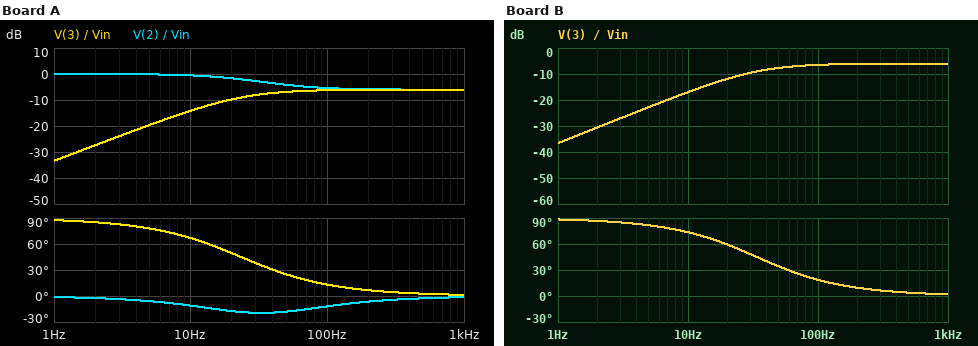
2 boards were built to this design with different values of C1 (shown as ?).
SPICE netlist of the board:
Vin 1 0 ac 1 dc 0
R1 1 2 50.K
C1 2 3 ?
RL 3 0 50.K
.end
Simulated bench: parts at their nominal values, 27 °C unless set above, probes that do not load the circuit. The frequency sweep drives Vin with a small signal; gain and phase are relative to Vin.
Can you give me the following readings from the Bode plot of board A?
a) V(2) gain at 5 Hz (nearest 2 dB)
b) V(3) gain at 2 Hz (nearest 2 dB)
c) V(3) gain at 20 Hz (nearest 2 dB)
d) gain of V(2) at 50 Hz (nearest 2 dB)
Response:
0 dB
-28 dB
-10 dB
-4 dB
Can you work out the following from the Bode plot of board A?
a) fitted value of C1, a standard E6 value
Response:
68 nF
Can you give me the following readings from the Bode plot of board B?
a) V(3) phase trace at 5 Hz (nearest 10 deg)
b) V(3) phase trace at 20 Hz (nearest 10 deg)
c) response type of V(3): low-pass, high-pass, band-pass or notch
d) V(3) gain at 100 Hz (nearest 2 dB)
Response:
80 deg
60 deg
high-pass
-6 dB
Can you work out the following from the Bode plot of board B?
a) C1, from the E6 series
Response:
47 nF
